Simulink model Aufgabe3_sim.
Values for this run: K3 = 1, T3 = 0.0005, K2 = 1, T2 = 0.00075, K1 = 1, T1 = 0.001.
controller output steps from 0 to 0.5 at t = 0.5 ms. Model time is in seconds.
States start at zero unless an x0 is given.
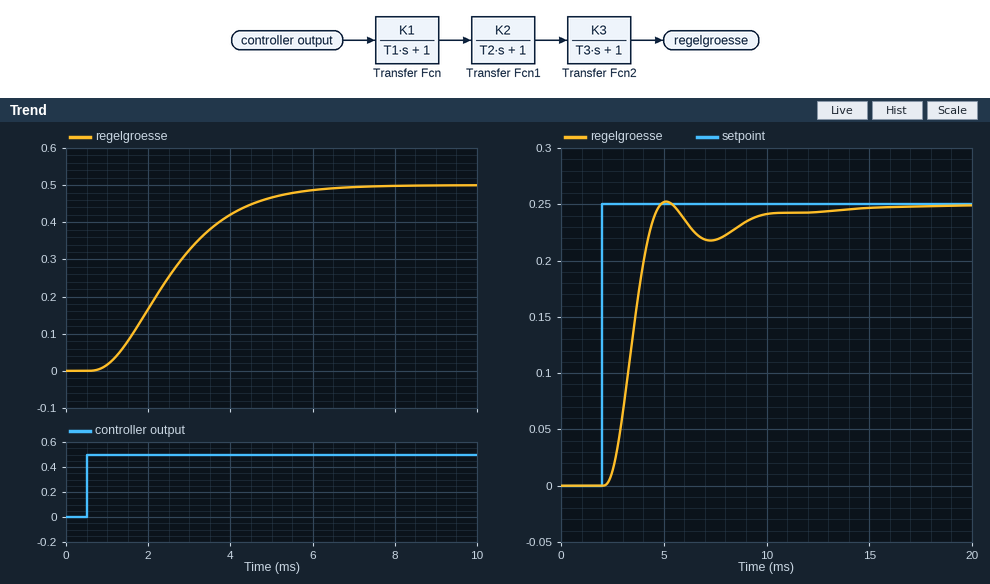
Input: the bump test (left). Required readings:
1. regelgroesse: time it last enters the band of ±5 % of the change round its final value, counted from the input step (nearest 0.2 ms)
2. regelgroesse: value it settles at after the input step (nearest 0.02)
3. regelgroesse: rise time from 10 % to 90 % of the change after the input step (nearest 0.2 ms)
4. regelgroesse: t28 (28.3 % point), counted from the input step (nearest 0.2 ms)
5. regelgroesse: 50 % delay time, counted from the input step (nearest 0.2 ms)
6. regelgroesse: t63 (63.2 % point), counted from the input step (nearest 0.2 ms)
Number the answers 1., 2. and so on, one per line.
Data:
1. 4.8 ms
2. 0.50
3. 3.2 ms
4. 1.4 ms
5. 2.0 ms
6. 2.4 ms
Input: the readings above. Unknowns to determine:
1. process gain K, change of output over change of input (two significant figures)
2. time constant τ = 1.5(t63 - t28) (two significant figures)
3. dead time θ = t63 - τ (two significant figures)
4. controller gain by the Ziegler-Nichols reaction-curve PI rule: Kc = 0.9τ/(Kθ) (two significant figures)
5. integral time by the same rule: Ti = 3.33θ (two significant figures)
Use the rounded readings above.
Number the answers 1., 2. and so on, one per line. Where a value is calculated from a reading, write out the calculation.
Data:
1. (0.5 - 0) / 0.5 = 1.0
2. 1.5 × (2.4 - 1.4) = 1.5 ms
3. 2.4 - 1.5 = 0.90 ms
4. 0.9 × 1.5 / (1 × 0.9) = 1.5
5. 3.33 × 0.9 = 3.0 ms
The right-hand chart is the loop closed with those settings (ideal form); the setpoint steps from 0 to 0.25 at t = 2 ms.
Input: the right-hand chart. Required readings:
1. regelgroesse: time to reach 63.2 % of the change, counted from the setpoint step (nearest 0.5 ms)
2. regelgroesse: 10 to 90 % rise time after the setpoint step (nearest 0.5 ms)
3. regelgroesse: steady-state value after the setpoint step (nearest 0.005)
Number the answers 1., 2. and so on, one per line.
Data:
1. 1.5 ms
2. 1.5 ms
3. 0.250
